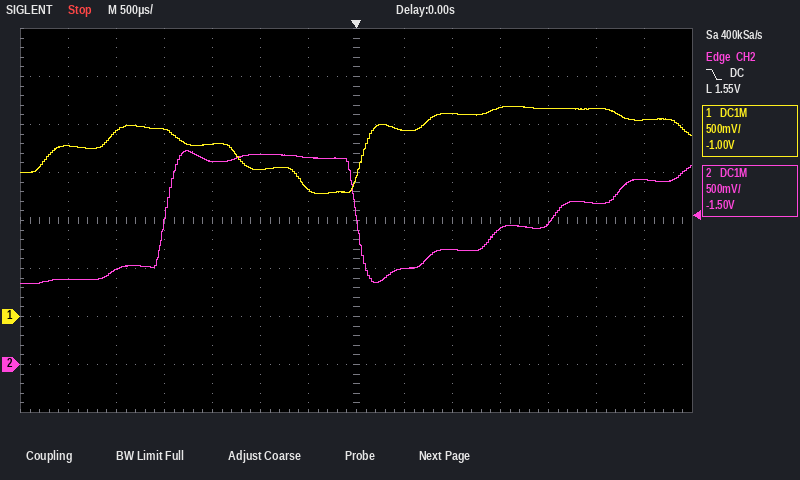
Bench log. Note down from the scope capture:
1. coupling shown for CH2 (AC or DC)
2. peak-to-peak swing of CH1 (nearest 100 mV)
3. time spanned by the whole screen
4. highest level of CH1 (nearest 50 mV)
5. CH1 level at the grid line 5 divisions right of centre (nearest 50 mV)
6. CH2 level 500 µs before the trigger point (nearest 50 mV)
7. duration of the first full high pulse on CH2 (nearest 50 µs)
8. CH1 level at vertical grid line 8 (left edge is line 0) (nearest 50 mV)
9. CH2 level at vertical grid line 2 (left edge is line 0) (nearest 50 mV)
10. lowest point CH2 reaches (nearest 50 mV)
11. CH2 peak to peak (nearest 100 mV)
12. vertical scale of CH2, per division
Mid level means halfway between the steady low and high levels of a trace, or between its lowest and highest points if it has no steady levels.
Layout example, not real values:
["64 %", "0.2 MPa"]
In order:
["DC", "900 mV", "7 ms", "2.20 V", "2.15 V", "2.15 V", "2.00 ms", "1.95 V", "1.00 V", "850 mV", "1.40 V", "500 mV"]
